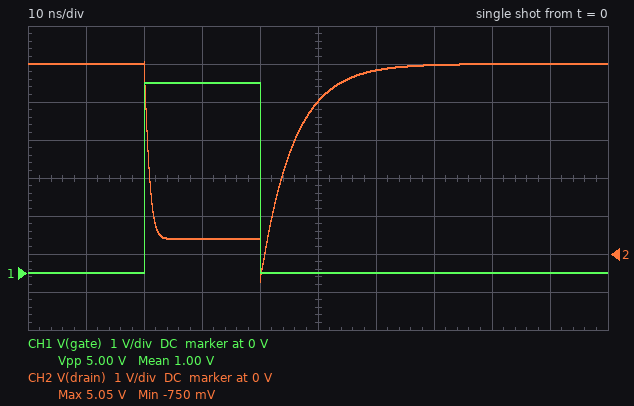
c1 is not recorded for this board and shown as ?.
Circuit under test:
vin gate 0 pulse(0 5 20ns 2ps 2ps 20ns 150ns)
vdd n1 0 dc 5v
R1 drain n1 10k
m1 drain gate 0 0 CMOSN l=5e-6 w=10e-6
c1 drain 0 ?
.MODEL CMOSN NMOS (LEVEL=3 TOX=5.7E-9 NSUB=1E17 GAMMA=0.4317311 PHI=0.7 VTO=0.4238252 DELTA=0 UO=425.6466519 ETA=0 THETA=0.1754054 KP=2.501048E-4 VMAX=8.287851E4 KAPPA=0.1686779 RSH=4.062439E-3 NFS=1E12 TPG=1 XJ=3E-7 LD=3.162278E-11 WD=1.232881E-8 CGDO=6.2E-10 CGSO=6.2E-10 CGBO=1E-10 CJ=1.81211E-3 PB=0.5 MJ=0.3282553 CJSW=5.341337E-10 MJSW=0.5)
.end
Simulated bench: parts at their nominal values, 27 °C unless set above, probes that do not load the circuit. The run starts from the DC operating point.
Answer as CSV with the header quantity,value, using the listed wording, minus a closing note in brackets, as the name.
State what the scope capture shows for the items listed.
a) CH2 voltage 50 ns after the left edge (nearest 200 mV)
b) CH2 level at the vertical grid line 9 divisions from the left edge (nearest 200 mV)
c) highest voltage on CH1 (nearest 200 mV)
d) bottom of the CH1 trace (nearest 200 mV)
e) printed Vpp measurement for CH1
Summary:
quantity,value
CH2 voltage 50 ns after the left edge,4.0 V
CH2 level at the vertical grid line 9 divisions from the left edge,5.0 V
highest voltage on CH1,5.0 V
bottom of the CH1 trace,0 V
printed Vpp measurement for CH1,5.00 V
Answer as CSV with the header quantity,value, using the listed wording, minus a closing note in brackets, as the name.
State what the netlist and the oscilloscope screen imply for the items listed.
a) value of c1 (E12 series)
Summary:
quantity,value
value of c1,560 fF
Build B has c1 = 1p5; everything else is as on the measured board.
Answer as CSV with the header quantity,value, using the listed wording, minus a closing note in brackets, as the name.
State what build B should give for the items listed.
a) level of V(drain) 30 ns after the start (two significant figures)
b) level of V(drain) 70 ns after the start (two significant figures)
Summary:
quantity,value
level of V(drain) 30 ns after the start,400 mV
level of V(drain) 70 ns after the start,4.3 V
